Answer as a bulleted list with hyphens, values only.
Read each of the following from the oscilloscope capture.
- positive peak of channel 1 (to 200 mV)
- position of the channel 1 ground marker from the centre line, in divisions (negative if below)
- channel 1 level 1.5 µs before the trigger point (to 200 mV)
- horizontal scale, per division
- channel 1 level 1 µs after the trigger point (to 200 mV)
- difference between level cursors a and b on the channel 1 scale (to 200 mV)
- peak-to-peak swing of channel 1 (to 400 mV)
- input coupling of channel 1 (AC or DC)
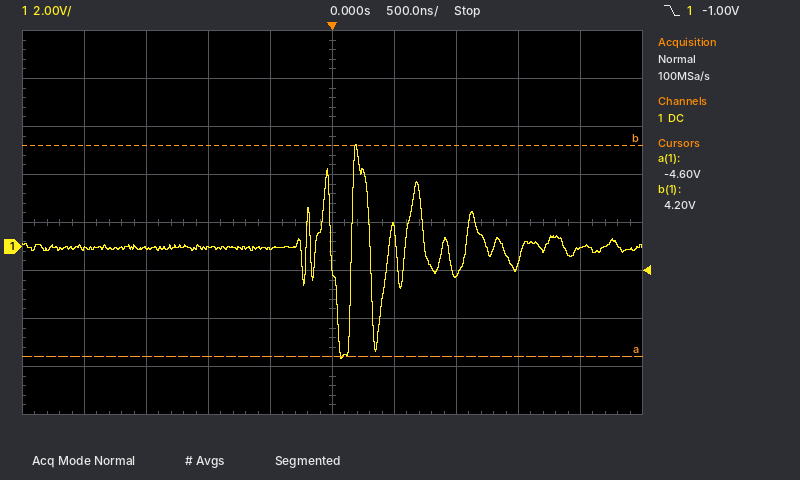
- 4.2 V
- -0.5 div
- 0.0 V
- 500 ns
- -1.2 V
- 8.8 V
- 8.8 V
- DC
